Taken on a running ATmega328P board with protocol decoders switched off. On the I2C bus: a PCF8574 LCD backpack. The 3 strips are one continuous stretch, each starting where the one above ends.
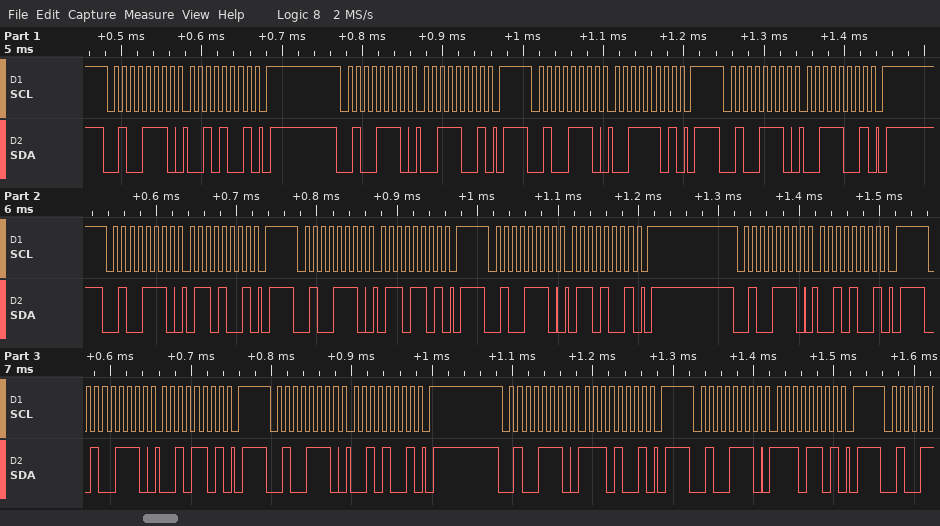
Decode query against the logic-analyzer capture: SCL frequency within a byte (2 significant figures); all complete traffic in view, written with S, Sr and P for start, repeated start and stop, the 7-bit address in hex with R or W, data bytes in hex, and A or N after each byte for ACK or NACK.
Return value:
100 kHz
S 27W A 29 A P S 27W A 39 A P S 27W A 3D A P S 27W A 39 A P S 27W A 69 A P S 27W A 6D A P S 27W A 69 A P S 27W A 29 A P S 27W A 2D A P S 27W A 29 A P S 27W A E9 A P S 27W A ED A P
